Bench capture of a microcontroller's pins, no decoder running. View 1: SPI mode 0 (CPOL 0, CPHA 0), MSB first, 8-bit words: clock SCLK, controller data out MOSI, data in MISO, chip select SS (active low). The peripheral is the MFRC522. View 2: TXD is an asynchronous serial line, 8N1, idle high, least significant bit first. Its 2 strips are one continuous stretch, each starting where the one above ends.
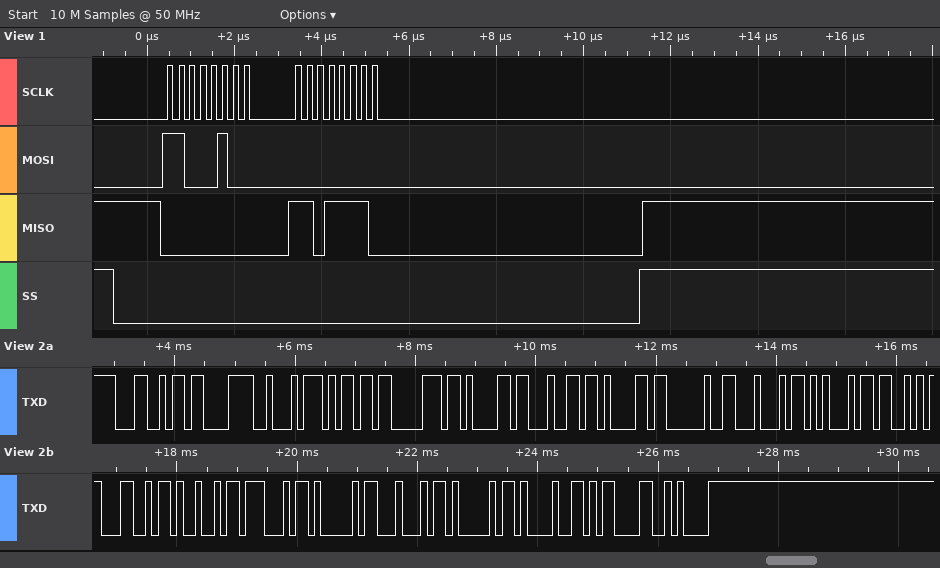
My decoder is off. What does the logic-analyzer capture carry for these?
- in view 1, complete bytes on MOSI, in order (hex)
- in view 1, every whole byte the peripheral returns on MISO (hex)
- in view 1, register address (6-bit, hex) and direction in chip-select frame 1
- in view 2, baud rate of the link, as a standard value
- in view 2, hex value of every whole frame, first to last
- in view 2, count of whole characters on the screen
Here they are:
C4 00
00 DE
0x22 read
9600 baud
4C C3 A2 6D 70 61 64 61 20 44 45 53 4C 49 47 41 44 41 21 0D 0A
21
